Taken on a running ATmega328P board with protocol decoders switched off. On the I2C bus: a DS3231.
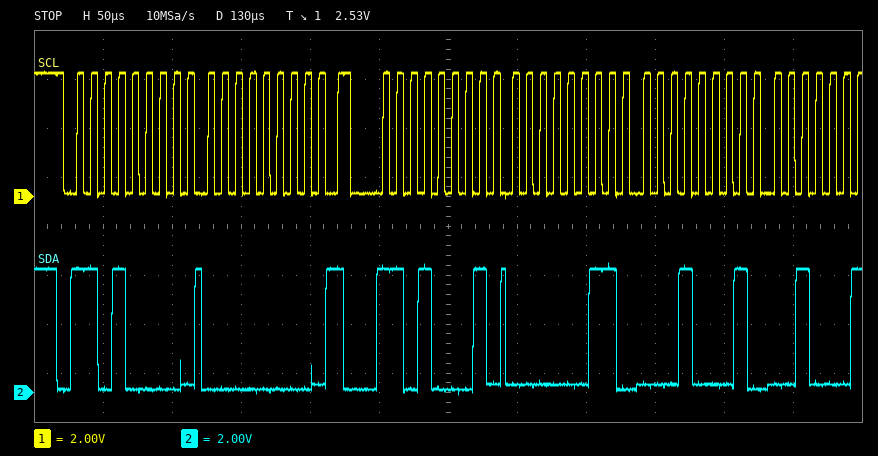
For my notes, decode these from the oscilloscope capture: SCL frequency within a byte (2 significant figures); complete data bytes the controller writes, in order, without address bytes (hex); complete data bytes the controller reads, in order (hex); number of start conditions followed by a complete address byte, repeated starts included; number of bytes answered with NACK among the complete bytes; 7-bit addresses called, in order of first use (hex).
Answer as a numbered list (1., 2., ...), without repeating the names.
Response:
1. 100 kHz
2. 00
3. 03 11
4. 2
5. 0
6. 0x68
